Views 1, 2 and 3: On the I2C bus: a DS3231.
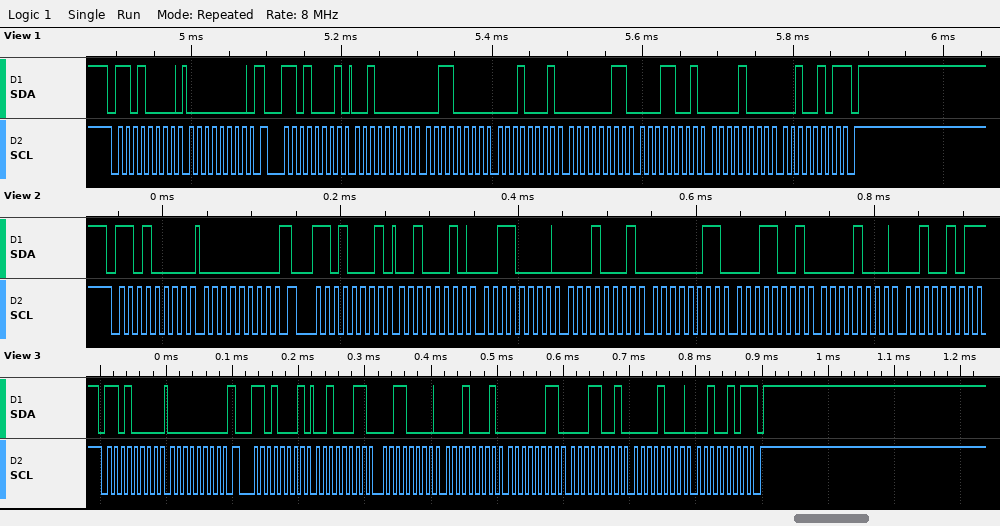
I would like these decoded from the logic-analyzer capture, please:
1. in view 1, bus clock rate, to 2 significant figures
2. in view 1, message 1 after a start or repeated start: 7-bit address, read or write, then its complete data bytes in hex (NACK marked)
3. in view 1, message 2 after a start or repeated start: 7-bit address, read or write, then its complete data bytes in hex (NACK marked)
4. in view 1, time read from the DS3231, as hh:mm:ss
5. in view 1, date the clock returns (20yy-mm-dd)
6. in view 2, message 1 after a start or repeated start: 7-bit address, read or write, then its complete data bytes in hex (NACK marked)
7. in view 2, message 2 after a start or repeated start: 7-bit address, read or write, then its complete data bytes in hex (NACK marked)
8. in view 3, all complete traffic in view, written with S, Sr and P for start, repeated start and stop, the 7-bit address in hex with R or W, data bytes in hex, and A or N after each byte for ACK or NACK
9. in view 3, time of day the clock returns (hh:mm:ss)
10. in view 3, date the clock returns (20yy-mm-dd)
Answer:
100 kHz
0x68 write: 00
0x68 read: 20 30 11 03 19 08 25 NACK
11:30:20
2025-08-19
0x68 write: 00
0x68 read: 22 30 11 03 19 08 25 NACK
S 68W A 00 A Sr 68R A 23 A 30 A 11 A 03 A 19 A 08 A 25 N P
11:30:23
2025-08-19
